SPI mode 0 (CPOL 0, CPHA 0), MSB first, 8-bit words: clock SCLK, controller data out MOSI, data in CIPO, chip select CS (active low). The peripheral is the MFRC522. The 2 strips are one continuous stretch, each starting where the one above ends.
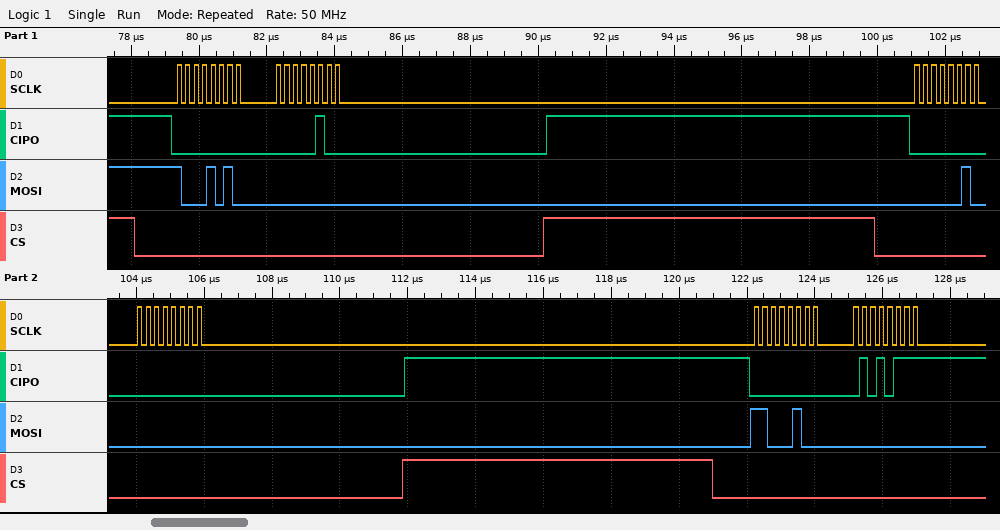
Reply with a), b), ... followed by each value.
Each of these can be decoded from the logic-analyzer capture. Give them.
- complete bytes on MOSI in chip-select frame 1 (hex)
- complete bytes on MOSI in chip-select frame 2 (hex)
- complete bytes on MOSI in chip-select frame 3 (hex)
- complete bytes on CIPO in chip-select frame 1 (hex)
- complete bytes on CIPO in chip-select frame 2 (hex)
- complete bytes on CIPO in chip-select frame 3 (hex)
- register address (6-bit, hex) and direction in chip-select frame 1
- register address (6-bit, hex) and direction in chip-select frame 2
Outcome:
a) 0x8A 0x00
b) 0x02 0x00
c) 0xC4 0x00
d) 0x00 0x04
e) 0x00 0x00
f) 0x00 0x57
g) 0x05 read
h) 0x01 write
